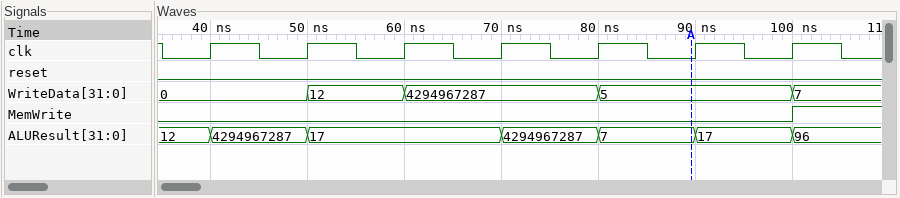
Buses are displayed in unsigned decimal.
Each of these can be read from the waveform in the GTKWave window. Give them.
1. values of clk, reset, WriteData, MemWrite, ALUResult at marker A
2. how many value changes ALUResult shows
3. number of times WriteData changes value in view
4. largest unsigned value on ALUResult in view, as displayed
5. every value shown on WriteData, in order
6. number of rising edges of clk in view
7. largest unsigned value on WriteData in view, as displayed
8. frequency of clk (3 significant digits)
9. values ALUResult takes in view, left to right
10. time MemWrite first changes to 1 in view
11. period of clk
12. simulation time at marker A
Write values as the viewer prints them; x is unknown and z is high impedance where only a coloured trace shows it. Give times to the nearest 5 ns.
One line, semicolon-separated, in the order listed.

clk=0, reset=0, WriteData=5, MemWrite=0, ALUResult=7; 6; 4; 4294967287; 0, 12, 4294967287, 5, 7; 7; 4294967287; 100 MHz; 12, 4294967287, 17, 4294967287, 7, 17, 96; 100 ns; 10 ns; 90 ns
